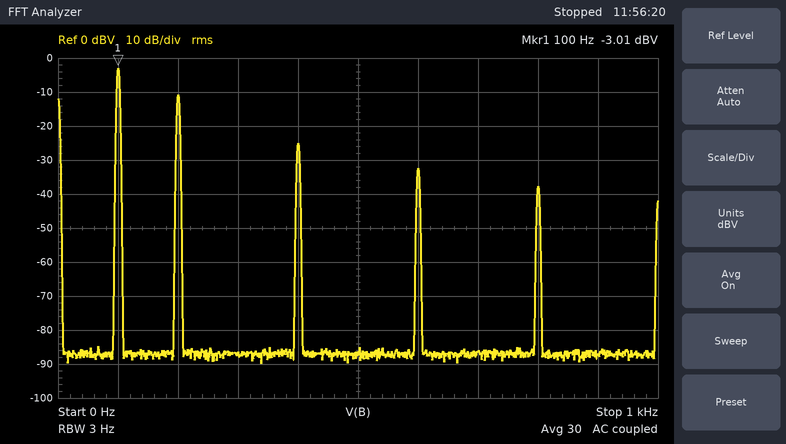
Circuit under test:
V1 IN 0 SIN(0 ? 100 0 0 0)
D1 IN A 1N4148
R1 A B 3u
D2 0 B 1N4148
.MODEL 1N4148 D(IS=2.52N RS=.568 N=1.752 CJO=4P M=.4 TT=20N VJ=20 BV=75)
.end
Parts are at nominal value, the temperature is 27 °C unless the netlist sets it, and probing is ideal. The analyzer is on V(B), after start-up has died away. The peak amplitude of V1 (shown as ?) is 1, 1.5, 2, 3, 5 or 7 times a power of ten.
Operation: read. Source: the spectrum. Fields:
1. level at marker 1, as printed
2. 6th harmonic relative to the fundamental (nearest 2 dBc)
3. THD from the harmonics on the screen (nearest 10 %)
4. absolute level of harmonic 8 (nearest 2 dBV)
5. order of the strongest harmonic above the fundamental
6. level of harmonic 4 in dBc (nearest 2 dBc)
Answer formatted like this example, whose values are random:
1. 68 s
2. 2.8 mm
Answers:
1. -3.01 dBV
2. -30 dBc
3. 40 %
4. -38 dBV
5. 2
6. -22 dBc
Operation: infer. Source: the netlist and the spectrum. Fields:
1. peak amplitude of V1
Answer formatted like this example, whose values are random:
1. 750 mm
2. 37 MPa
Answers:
1. 2 V
